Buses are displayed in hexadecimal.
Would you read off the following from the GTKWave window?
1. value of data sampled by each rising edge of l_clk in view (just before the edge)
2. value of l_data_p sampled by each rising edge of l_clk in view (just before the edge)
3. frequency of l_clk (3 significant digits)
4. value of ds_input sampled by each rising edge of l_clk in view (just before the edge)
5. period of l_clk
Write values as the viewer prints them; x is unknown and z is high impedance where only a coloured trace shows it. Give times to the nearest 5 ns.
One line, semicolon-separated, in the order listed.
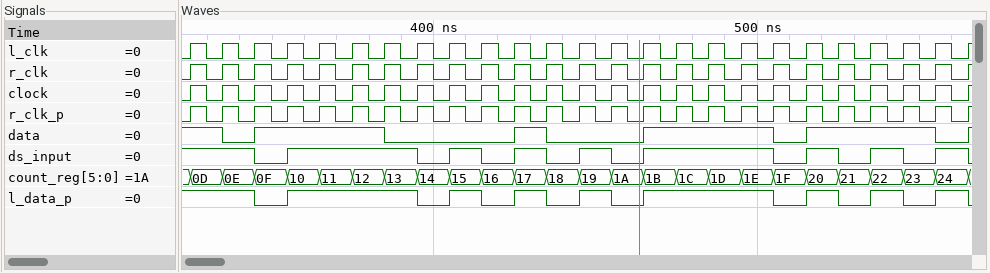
1 1 0 1 1 1 1 0 0 0 0 1 0 0 0 1 1 1 1 0 1 1 1 1 0; 1 1 1 0 1 1 1 1 0 1 0 1 0 1 0 1 1 1 1 0 1 0 1 0 1; 100 MHz; 1 1 1 0 1 1 1 1 0 1 0 1 0 1 0 1 1 1 1 0 1 0 1 0 1; 10 ns
